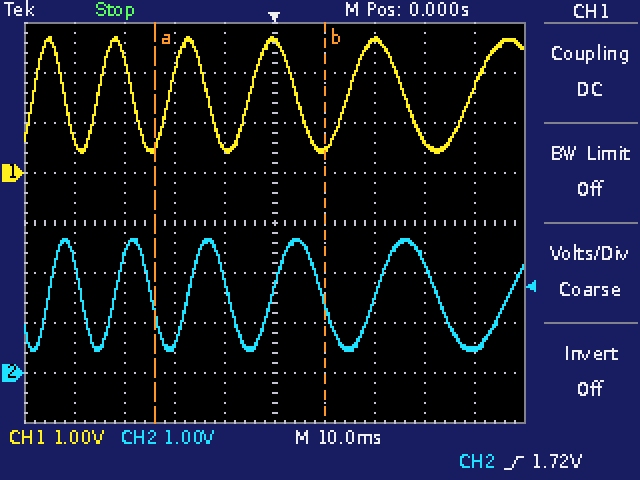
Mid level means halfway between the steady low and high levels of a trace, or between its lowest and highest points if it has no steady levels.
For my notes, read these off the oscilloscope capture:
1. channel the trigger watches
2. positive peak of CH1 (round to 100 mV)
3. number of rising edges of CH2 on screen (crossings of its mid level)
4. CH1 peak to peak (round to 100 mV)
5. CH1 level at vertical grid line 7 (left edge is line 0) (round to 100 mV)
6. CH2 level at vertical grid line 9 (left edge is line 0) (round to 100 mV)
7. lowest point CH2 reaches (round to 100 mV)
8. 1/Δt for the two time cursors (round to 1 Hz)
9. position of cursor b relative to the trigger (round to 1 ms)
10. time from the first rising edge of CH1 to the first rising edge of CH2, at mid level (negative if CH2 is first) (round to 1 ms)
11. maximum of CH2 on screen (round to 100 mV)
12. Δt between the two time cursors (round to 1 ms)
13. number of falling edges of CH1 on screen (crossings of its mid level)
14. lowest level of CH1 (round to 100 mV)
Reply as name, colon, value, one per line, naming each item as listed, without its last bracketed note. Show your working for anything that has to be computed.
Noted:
channel the trigger watches: CH2
positive peak of CH1: 2.7 V
number of rising edges of CH2 on screen: 6
CH1 peak to peak: 2.7 V − (400 mV) = 2.3 V
CH1 level at vertical grid line 7 (left edge is line 0): 2.7 V
CH2 level at vertical grid line 9 (left edge is line 0): 500 mV
lowest point CH2 reaches: 400 mV
1/Δt for the two time cursors: 1 / 34 ms ≈ 29 Hz
position of cursor b relative to the trigger: +10 ms
time from the first rising edge of CH1 to the first rising edge of CH2, at mid level (negative if CH2 is first): +3 ms
maximum of CH2 on screen: 2.7 V
Δt between the two time cursors: 34 ms
number of falling edges of CH1 on screen: 5
lowest level of CH1: 400 mV
